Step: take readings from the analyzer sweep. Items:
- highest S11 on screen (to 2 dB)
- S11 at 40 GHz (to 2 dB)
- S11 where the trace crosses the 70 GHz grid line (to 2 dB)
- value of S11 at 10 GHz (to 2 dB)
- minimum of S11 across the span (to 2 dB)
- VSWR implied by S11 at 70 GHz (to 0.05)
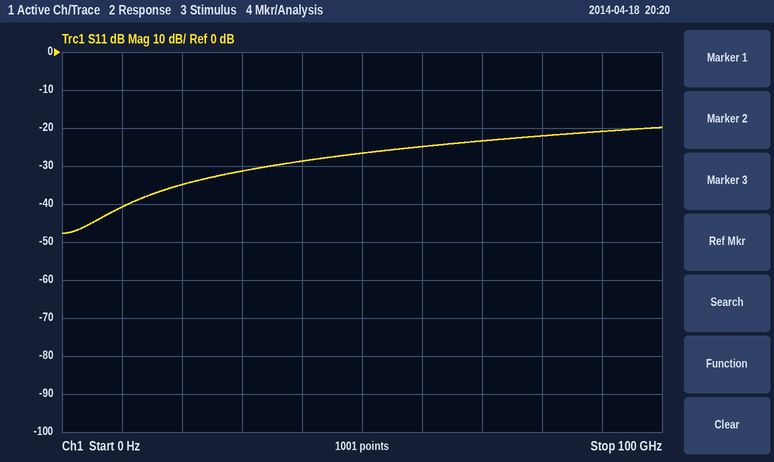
-20 dB
-28 dB
-24 dB
-40 dB
-48 dB
1.15
